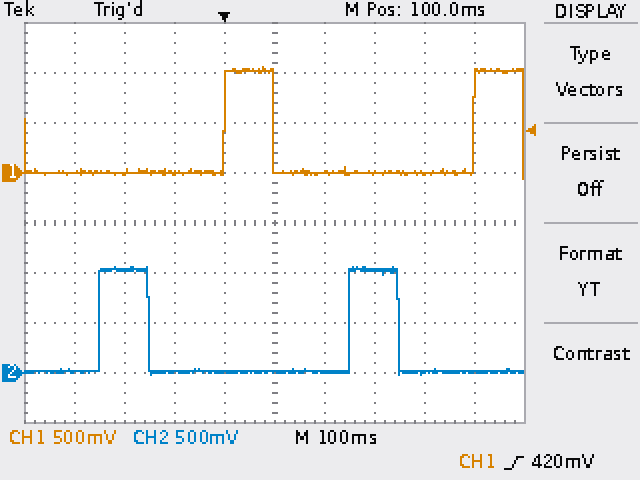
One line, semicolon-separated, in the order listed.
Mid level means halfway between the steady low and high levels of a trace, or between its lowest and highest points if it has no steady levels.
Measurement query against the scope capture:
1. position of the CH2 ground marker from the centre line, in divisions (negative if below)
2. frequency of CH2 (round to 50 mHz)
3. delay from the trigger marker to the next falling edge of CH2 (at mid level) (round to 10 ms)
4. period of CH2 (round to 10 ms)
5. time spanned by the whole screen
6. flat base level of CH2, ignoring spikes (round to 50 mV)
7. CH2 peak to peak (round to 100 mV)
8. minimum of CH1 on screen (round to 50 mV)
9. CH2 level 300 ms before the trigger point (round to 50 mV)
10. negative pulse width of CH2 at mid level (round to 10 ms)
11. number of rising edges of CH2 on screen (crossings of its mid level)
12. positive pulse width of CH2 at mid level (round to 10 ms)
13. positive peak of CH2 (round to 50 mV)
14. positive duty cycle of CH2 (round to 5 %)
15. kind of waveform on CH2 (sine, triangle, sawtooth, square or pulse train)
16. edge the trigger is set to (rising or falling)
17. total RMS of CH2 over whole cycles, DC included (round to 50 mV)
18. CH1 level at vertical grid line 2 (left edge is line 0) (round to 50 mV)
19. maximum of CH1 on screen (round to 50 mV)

-3.0 div; 2.00 Hz; 350 ms; 500 ms; 1 s; 0 mV; 1.10 V; -50 mV; 0 mV; 400 ms; 2; 100 ms; 1.05 V; 20 %; pulse train; rising; 450 mV; 0 mV; 1.05 V
